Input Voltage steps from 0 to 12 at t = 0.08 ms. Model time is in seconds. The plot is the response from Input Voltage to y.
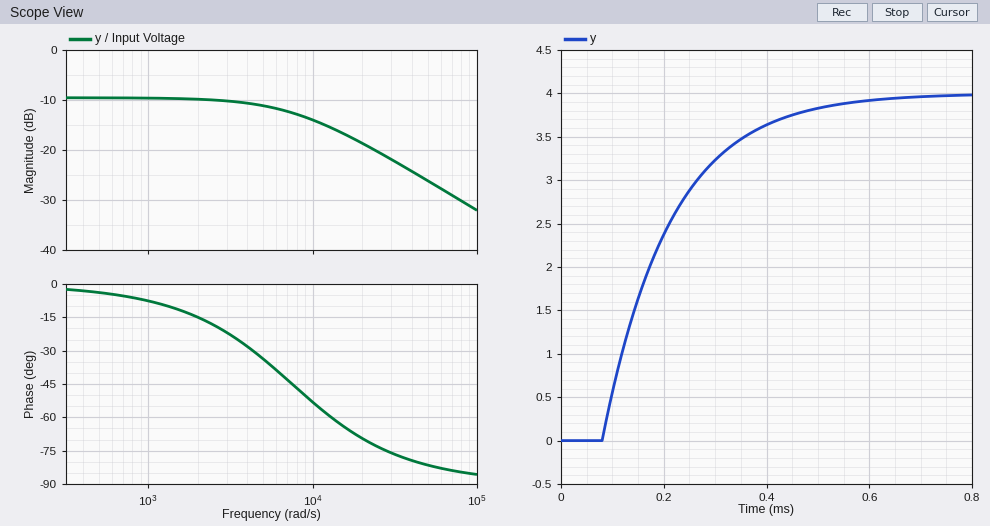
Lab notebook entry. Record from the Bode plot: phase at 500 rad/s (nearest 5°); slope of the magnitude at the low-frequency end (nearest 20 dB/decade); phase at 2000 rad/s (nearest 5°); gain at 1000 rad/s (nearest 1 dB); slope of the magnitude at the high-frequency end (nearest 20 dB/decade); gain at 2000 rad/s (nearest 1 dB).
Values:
-5°
0 dB/decade
-15°
-10 dB
-20 dB/decade
-10 dB
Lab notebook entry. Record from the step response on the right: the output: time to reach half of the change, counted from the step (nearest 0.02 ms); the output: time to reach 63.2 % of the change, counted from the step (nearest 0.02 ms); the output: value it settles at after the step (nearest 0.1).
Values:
0.10 ms
0.14 ms
4.0
